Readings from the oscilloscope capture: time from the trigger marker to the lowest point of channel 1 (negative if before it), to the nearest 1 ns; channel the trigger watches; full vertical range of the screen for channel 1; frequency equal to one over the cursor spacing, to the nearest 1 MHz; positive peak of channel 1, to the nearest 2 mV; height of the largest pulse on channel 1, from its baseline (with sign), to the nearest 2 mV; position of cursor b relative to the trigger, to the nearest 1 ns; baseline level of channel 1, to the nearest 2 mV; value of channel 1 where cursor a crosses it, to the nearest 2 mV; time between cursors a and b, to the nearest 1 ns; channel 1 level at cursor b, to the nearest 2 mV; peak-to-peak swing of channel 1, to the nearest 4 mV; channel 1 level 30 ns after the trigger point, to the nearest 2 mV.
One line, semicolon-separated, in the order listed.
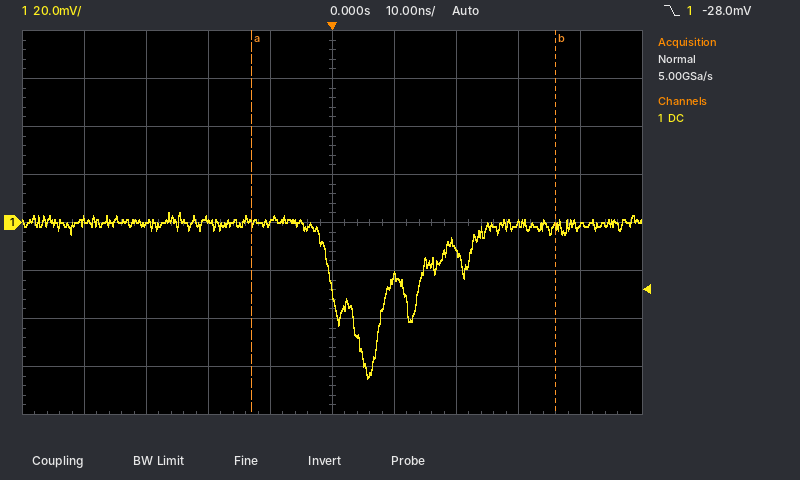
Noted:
+6 ns; channel 1; 160 mV; 20 MHz; 4 mV; -64 mV; +36 ns; 0 mV; 0 mV; 49 ns; -2 mV; 68 mV; 0 mV
